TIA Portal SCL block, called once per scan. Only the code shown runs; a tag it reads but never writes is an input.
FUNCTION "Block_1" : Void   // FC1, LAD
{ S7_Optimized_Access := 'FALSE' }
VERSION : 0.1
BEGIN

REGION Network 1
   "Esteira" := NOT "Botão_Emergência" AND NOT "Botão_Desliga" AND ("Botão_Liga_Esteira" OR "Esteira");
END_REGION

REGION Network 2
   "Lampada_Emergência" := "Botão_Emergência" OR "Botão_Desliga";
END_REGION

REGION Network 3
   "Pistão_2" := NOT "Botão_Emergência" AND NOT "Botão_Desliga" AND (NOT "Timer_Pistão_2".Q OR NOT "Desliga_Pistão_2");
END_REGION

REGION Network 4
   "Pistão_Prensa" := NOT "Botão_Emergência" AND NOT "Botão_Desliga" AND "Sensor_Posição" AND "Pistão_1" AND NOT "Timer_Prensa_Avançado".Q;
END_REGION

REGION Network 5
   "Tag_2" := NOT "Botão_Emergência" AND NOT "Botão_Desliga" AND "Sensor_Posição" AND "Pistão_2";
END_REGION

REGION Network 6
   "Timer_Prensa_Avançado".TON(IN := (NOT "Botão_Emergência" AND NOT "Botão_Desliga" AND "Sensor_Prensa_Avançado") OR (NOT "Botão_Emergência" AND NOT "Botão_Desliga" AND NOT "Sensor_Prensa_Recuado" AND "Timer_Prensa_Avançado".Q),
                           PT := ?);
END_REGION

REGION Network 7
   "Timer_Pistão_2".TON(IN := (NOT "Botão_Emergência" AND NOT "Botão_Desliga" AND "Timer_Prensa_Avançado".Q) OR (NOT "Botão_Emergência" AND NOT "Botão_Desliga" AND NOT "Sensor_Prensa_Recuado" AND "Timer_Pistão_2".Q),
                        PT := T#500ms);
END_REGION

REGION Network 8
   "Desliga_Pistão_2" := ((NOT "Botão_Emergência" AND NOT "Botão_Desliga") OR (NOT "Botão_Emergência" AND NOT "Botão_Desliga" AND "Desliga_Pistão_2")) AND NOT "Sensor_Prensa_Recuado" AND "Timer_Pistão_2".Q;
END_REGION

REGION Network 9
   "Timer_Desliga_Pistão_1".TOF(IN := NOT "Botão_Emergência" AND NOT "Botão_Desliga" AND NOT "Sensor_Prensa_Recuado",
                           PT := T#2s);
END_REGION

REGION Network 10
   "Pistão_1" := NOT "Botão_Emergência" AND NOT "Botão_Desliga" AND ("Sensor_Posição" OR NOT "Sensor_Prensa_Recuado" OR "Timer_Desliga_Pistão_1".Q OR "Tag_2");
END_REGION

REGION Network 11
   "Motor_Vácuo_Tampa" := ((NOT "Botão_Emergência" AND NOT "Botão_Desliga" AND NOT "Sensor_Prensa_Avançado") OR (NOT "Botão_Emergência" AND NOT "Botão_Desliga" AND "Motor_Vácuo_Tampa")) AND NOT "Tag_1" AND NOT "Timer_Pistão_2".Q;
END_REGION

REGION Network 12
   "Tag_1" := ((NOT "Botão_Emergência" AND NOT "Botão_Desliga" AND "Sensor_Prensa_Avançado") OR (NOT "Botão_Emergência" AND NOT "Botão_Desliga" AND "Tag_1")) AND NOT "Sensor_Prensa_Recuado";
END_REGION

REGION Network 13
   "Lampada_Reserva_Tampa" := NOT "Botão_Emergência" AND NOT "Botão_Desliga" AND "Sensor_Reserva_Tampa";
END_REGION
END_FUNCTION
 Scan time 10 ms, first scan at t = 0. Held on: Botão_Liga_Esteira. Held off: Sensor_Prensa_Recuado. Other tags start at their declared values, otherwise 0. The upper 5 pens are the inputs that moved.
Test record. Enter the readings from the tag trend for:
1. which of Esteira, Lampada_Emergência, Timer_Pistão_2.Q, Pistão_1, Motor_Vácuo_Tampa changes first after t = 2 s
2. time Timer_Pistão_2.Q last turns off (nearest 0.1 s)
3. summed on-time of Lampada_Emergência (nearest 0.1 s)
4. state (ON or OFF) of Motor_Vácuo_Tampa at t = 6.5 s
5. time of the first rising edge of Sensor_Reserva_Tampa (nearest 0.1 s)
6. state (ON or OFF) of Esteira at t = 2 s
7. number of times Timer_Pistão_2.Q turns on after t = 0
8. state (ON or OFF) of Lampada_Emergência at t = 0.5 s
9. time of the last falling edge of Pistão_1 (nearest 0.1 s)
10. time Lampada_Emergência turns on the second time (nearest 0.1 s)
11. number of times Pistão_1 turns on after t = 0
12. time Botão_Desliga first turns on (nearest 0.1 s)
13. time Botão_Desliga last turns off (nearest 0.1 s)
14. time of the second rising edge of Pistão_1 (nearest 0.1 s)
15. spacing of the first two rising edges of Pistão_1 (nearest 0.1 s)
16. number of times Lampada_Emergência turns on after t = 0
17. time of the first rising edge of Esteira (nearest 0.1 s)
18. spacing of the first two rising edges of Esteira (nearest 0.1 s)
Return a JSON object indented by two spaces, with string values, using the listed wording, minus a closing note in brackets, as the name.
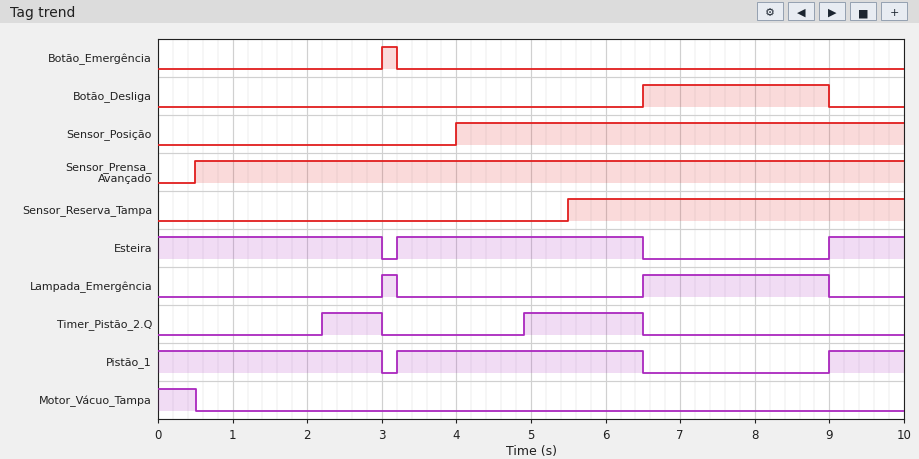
{
  "which of Esteira, Lampada_Emergência, Timer_Pistão_2.Q, Pistão_1, Motor_Vácuo_Tampa changes first after t = 2 s": "Timer_Pistão_2.Q",
  "time Timer_Pistão_2.Q last turns off": "6.5 s",
  "summed on-time of Lampada_Emergência": "2.7 s",
  "state (ON or OFF) of Motor_Vácuo_Tampa at t = 6.5 s": "OFF",
  "time of the first rising edge of Sensor_Reserva_Tampa": "5.5 s",
  "state (ON or OFF) of Esteira at t = 2 s": "ON",
  "number of times Timer_Pistão_2.Q turns on after t = 0": "2",
  "state (ON or OFF) of Lampada_Emergência at t = 0.5 s": "OFF",
  "time of the last falling edge of Pistão_1": "6.5 s",
  "time Lampada_Emergência turns on the second time": "6.5 s",
  "number of times Pistão_1 turns on after t = 0": "2",
  "time Botão_Desliga first turns on": "6.5 s",
  "time Botão_Desliga last turns off": "9.0 s",
  "time of the second rising edge of Pistão_1": "9.0 s",
  "spacing of the first two rising edges of Pistão_1": "5.8 s",
  "number of times Lampada_Emergência turns on after t = 0": "2",
  "time of the first rising edge of Esteira": "3.2 s",
  "spacing of the first two rising edges of Esteira": "5.8 s"
}
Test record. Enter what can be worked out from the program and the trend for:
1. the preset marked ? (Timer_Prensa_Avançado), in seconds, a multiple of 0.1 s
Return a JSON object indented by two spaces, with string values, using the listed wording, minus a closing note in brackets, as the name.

{
  "the preset marked ? (Timer_Prensa_Avançado), in seconds, a multiple of 0.1 s": "1.2 s"
}
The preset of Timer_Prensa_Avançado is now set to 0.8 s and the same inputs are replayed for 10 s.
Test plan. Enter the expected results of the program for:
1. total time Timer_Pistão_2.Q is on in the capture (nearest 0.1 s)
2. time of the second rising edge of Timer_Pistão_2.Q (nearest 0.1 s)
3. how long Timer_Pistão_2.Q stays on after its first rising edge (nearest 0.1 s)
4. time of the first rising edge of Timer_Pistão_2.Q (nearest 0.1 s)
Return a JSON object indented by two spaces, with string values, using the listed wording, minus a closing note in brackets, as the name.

{
  "total time Timer_Pistão_2.Q is on in the capture": "3.2 s",
  "time of the second rising edge of Timer_Pistão_2.Q": "4.5 s",
  "how long Timer_Pistão_2.Q stays on after its first rising edge": "1.2 s",
  "time of the first rising edge of Timer_Pistão_2.Q": "1.8 s"
}
